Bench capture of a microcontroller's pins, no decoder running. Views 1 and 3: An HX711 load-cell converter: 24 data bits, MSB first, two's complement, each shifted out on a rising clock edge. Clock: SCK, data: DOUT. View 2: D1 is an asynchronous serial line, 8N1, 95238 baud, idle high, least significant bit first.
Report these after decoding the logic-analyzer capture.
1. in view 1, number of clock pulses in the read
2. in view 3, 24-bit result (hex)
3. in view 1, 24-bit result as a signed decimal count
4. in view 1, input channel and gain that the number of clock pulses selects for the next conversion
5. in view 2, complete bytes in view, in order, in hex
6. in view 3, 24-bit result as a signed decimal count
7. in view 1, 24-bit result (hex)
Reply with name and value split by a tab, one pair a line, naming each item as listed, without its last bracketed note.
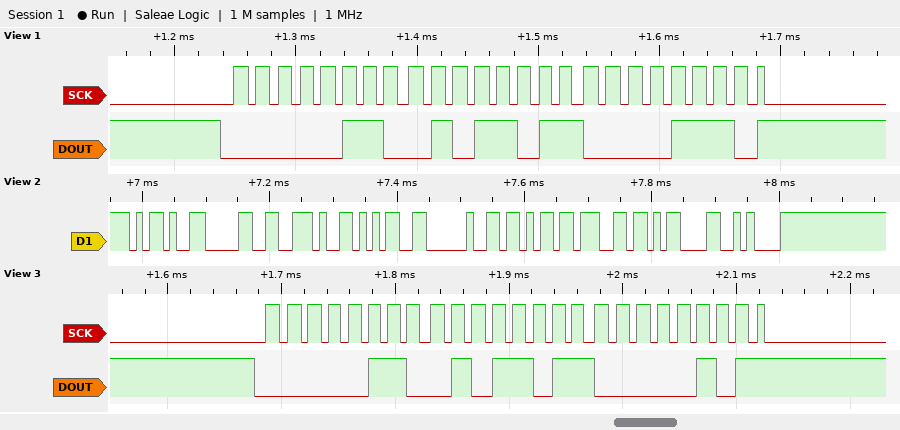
in view 1, number of clock pulses in the read	25
in view 3, 24-bit result	0x065B05
in view 1, 24-bit result as a signed decimal count	416526
in view 1, input channel and gain that the number of clock pulses selects for the next conversion	channel A, gain 128
in view 2, complete bytes in view, in order, in hex	0x2D 0x30 0x2E 0x35 0x20 0x6B 0x67 0x0D 0x0A
in view 3, 24-bit result as a signed decimal count	416517
in view 1, 24-bit result	0x065B0E
